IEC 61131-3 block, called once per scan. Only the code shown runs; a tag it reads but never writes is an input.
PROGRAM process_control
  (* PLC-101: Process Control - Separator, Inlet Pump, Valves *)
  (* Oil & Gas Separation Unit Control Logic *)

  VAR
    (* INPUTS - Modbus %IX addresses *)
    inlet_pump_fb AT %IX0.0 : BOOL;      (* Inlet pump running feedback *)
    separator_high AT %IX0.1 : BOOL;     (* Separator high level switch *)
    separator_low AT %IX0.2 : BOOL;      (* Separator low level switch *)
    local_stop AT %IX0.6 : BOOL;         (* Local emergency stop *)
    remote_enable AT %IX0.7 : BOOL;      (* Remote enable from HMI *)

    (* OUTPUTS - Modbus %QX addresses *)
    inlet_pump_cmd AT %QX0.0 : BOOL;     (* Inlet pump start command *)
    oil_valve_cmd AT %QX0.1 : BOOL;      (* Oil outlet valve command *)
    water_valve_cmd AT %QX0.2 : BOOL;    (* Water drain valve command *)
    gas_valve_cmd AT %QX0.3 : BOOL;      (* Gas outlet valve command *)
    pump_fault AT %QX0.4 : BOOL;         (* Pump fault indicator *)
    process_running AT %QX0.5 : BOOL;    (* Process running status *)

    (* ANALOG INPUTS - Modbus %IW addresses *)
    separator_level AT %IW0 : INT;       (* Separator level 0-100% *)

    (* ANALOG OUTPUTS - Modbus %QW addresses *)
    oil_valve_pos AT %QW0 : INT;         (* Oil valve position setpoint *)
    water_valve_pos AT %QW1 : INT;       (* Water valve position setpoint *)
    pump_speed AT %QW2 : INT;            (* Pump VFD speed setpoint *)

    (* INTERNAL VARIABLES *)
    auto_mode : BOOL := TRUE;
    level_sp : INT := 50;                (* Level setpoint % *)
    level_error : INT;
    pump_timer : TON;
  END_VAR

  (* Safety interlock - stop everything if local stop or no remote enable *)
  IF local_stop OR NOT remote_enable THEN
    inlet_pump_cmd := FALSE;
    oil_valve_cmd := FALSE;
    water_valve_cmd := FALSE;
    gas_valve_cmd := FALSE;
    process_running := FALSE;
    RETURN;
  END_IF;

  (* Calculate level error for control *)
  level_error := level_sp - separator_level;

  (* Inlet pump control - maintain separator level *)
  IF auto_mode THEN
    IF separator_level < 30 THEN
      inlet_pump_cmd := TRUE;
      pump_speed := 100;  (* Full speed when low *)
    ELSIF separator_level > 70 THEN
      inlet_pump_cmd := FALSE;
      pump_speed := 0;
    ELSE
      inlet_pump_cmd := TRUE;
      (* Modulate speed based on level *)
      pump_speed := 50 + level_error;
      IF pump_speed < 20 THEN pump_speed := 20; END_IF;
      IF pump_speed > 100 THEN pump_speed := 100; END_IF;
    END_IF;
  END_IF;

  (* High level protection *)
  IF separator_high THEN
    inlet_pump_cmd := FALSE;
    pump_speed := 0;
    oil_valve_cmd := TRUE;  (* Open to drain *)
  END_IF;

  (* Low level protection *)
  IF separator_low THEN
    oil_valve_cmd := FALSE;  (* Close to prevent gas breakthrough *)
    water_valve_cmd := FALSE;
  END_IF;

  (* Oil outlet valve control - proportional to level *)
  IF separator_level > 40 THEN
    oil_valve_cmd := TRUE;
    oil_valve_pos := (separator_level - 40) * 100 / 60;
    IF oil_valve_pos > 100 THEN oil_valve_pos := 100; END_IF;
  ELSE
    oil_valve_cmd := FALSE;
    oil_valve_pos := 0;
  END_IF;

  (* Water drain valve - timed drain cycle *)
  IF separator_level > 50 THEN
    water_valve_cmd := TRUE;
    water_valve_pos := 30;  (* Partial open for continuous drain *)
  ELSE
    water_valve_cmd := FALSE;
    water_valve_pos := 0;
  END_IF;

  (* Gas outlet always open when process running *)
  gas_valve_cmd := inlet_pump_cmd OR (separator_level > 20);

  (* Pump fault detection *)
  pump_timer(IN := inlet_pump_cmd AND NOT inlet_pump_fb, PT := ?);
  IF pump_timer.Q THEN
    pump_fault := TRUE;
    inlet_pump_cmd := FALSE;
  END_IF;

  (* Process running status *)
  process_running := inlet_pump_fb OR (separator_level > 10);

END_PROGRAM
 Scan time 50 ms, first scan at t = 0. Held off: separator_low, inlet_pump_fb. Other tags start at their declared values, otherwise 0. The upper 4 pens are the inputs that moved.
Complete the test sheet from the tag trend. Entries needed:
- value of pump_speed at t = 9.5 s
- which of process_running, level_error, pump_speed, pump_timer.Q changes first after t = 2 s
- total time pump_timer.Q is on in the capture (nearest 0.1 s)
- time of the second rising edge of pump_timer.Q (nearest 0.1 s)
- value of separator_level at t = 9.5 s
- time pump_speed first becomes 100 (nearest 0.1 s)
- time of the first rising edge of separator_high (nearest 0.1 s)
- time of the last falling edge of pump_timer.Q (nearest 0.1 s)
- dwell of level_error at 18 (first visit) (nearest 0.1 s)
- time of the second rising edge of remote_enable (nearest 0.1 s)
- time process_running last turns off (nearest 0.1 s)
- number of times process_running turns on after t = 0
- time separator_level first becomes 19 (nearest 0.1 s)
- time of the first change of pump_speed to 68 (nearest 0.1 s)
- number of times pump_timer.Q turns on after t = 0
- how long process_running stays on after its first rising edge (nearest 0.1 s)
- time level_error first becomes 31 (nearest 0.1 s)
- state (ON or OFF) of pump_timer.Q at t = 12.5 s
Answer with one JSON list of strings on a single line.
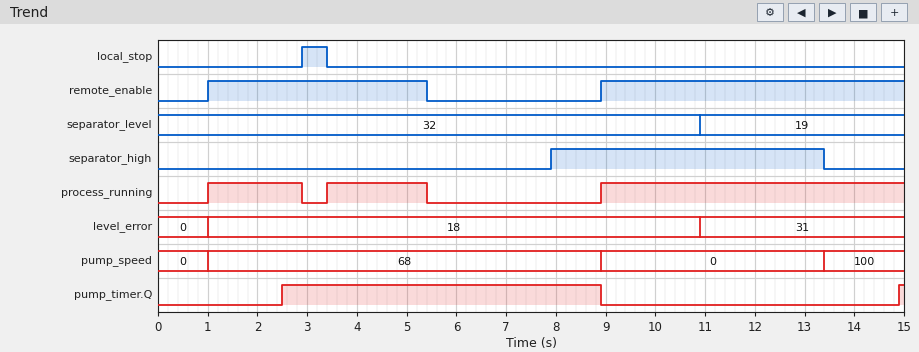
["0", "pump_timer.Q", "6.5 s", "14.9 s", "32", "13.4 s", "7.9 s", "8.9 s", "9.9 s", "8.9 s", "5.4 s", "3", "10.9 s", "1.0 s", "2", "1.9 s", "10.9 s", "OFF"]
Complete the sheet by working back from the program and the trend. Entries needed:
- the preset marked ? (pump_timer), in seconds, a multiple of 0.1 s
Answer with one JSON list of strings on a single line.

["1.5 s"]
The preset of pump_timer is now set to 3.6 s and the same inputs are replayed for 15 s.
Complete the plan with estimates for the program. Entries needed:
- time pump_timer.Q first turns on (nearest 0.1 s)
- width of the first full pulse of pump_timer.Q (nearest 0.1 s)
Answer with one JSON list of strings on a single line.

["4.6 s", "4.3 s"]
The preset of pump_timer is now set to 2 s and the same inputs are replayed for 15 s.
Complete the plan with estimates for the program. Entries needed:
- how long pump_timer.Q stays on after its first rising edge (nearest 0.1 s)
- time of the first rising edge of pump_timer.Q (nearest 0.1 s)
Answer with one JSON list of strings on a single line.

["5.5 s", "3.4 s"]
